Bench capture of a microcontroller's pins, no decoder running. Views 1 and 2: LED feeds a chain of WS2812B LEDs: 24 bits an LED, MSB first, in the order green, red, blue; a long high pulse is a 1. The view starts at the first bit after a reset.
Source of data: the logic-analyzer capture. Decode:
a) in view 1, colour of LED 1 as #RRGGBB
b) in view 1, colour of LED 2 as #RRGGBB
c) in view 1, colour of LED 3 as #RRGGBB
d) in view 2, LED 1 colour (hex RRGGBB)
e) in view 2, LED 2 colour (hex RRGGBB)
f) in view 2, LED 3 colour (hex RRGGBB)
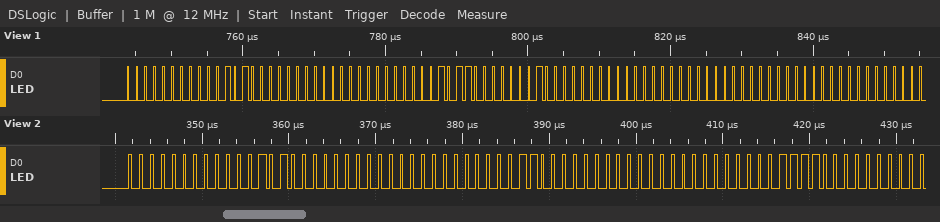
#140000
#160002
#000000
#0A0000
#0C0000
#0F0000
